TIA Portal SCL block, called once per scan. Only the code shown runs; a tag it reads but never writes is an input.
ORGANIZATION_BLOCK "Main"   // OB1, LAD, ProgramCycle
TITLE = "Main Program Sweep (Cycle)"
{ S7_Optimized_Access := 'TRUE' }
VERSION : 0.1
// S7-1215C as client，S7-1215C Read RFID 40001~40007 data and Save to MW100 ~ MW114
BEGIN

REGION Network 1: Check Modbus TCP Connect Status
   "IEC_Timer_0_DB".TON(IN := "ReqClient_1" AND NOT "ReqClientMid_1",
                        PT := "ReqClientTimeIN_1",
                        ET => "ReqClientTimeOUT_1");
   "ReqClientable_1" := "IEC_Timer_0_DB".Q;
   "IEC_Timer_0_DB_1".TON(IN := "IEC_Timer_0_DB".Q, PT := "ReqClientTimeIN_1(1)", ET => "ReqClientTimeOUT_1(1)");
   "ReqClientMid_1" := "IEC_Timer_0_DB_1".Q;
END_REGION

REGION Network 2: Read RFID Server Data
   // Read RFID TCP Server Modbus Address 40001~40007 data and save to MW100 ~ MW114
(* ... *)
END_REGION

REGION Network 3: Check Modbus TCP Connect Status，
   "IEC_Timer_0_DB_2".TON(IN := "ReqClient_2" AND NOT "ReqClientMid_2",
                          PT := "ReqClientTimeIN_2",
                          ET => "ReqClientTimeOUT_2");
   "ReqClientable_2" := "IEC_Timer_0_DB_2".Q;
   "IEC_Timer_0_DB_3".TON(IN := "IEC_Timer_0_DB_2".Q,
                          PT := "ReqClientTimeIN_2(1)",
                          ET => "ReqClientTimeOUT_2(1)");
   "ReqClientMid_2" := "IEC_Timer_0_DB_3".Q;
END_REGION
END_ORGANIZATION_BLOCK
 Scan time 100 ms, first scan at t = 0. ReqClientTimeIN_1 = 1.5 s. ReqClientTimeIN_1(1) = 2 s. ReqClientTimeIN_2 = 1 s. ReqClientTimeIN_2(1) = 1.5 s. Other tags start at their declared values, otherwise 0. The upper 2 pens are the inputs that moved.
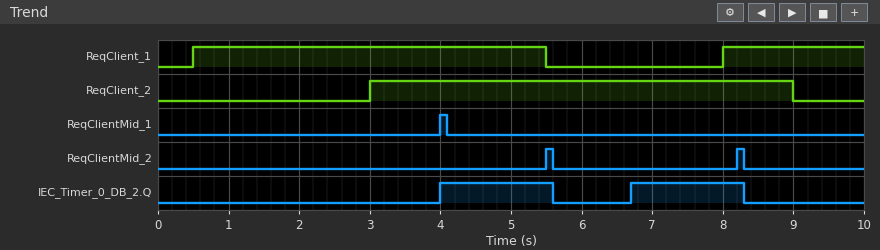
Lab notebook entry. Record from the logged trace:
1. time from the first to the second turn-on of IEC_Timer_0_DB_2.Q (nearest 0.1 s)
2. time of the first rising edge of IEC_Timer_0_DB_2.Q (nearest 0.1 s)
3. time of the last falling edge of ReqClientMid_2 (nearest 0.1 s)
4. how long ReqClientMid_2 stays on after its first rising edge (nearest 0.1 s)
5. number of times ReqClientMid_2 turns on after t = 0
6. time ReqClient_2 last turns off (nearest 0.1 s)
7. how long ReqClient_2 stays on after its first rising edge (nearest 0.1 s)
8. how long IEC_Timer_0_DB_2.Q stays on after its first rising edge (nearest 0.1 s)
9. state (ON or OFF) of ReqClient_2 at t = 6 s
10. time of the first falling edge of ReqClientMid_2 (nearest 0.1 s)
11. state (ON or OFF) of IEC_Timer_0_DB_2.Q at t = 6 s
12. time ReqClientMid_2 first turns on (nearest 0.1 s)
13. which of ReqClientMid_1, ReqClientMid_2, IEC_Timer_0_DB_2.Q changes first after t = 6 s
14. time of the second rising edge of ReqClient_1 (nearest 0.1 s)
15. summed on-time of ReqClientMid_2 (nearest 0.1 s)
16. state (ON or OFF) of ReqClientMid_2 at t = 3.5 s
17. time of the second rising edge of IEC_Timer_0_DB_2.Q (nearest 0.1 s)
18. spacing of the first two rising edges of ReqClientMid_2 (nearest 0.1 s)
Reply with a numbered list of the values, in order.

1. 2.7 s
2. 4.0 s
3. 8.3 s
4. 0.1 s
5. 2
6. 9.0 s
7. 6.0 s
8. 1.6 s
9. ON
10. 5.6 s
11. OFF
12. 5.5 s
13. IEC_Timer_0_DB_2.Q
14. 8.0 s
15. 0.2 s
16. OFF
17. 6.7 s
18. 2.7 s
